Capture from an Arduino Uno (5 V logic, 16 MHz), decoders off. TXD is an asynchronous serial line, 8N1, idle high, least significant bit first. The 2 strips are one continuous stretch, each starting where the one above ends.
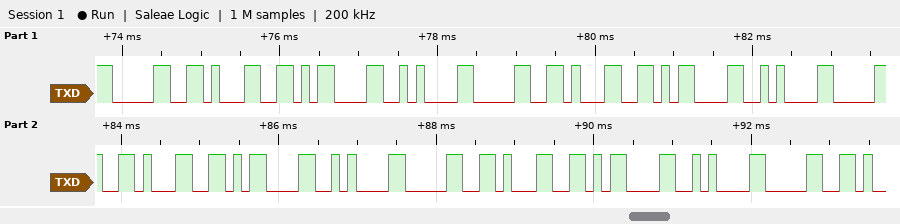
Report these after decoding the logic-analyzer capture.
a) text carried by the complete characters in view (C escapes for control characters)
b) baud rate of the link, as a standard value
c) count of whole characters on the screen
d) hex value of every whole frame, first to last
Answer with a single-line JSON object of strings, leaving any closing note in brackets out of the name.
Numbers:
{"text carried by the complete characters in view": "\"01\\r\\n01\\r\\n01\\r\\n01\\r\\n0\"", "baud rate of the link, as a standard value": "9600 baud", "count of whole characters on the screen": "17", "hex value of every whole frame, first to last": "0x30 0x31 0x0D 0x0A 0x30 0x31 0x0D 0x0A 0x30 0x31 0x0D 0x0A 0x30 0x31 0x0D 0x0A 0x30"}
